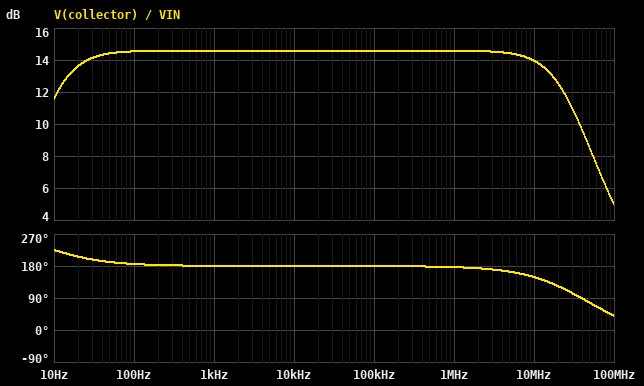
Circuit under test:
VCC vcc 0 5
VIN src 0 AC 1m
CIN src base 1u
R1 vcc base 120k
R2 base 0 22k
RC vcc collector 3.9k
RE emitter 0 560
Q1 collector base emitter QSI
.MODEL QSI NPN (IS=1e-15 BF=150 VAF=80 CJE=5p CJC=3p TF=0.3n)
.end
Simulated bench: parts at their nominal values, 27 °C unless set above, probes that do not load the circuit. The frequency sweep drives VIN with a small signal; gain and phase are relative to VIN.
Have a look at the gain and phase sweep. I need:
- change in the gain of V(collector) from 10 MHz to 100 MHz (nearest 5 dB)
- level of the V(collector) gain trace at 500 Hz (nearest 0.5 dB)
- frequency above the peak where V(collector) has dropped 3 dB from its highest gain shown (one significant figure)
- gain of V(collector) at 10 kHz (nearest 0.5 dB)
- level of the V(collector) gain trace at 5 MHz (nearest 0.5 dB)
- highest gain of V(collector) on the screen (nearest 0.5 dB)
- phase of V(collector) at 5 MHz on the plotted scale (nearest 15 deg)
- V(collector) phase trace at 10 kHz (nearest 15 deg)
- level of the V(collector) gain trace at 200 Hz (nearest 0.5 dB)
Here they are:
-10 dB
14.5 dB
30 MHz
14.5 dB
14.5 dB
14.5 dB
165 deg
180 deg
14.5 dB
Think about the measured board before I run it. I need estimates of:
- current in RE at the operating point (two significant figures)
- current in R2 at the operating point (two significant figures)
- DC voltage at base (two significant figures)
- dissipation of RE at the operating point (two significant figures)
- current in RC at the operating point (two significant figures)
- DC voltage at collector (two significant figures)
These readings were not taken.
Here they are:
160 µA
34 µA
760 mV
14 µW
160 µA
4.4 V
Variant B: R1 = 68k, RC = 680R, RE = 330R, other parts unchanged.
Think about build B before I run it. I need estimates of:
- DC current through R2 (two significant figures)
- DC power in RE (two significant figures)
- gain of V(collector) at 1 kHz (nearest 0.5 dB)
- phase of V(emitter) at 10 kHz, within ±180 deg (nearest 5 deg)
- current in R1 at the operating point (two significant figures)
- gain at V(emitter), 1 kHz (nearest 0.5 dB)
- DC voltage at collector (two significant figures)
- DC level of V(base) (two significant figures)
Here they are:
50 µA
440 µW
5.5 dB
0 deg
57 µA
-0.5 dB
4.2 V
1.1 V
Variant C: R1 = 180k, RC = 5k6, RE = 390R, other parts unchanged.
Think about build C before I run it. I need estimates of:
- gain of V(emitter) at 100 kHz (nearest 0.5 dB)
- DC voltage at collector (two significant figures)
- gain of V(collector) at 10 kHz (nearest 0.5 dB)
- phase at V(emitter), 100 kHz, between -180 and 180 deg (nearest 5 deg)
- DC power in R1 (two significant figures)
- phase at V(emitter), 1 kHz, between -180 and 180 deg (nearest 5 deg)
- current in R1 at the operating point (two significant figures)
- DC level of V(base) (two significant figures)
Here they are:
-33.5 dB
5.0 V
-10.5 dB
5 deg
110 µW
0 deg
25 µA
540 mV
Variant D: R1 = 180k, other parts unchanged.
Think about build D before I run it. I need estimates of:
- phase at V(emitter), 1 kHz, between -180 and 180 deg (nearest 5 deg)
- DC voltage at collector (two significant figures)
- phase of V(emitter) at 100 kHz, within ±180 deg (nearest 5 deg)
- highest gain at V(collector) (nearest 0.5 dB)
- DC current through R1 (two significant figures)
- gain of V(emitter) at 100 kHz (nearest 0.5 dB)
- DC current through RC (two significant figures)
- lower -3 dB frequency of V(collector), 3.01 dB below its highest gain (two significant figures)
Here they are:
0 deg
5.0 V
5 deg
0 dB
25 µA
-30.5 dB
1.4 µA
21 MHz
